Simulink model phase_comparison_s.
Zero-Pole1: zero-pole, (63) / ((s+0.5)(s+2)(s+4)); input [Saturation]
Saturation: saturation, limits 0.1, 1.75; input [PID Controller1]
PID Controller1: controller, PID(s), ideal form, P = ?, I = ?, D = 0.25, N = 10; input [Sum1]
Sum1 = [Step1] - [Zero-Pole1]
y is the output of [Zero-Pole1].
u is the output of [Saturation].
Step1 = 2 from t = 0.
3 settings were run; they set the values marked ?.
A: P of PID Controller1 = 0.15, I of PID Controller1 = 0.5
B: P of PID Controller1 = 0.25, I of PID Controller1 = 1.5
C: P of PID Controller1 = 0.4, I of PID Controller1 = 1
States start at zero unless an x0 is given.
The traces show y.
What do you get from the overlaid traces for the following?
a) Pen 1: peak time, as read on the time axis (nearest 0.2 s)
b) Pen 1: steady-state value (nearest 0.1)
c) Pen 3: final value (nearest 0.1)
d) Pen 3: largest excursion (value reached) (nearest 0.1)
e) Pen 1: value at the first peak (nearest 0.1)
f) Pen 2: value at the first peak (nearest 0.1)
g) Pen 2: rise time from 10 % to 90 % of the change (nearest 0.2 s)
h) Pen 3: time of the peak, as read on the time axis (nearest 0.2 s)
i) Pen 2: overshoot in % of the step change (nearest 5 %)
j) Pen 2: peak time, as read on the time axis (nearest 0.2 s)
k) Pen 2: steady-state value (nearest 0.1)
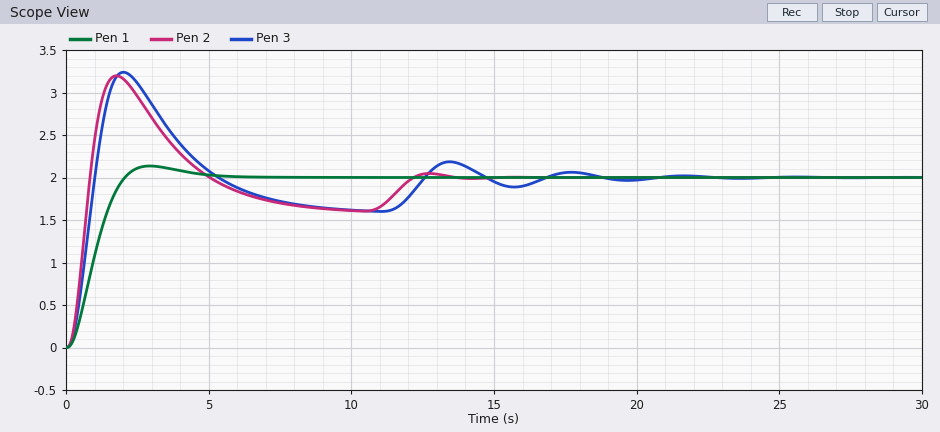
3.0 s
2.0
2.0
3.2
2.1
3.2
0.6 s
2.0 s
60 %
1.8 s
2.0
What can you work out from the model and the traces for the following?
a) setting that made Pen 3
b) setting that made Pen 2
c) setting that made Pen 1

B
C
A
